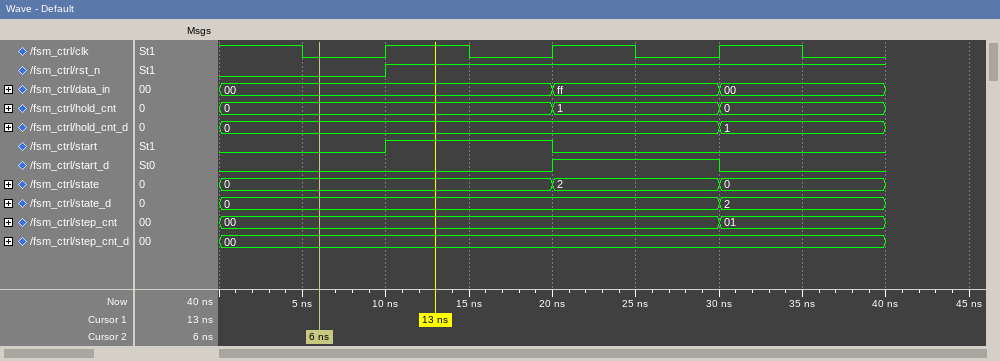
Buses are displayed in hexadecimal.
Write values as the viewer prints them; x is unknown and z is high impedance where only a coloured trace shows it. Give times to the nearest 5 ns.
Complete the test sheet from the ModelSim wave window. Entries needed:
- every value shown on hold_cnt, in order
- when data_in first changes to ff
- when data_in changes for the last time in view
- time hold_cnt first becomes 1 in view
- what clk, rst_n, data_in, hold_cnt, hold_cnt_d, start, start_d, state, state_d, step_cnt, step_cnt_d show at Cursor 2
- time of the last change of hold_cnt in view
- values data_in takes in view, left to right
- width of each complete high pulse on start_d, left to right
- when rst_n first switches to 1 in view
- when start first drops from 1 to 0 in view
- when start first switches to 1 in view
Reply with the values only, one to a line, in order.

0, 1, 0
20 ns
30 ns
20 ns
clk=0, rst_n=0, data_in=00, hold_cnt=0, hold_cnt_d=0, start=0, start_d=0, state=0, state_d=0, step_cnt=00, step_cnt_d=00
30 ns
00, ff, 00
10 ns
10 ns
20 ns
10 ns
